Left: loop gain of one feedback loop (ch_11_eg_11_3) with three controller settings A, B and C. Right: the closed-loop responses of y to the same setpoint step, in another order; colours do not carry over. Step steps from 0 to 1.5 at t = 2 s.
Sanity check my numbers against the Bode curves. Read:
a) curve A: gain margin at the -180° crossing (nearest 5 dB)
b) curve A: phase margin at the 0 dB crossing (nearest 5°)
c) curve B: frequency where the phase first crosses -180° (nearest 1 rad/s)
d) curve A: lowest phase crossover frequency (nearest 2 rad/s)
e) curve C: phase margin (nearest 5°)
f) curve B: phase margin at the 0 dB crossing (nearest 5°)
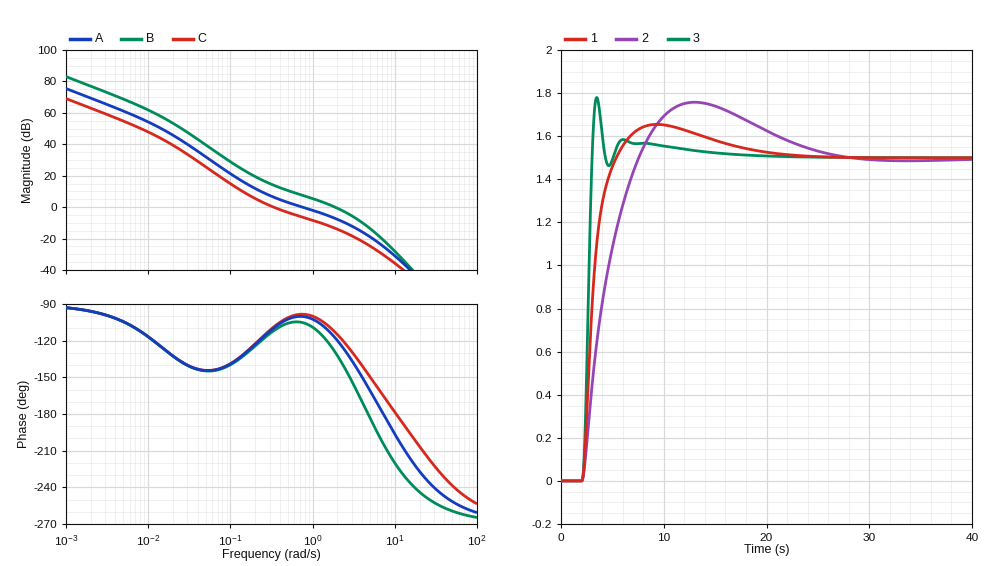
25 dB
80°
5 rad/s
8 rad/s
70°
50°
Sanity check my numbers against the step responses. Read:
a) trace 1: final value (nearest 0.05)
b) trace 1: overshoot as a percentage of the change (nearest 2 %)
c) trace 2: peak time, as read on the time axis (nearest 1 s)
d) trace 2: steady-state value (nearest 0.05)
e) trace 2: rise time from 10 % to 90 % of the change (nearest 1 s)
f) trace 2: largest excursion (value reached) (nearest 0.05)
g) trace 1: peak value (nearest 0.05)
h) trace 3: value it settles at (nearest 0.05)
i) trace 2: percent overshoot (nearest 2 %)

1.50
10 %
13 s
1.50
4 s
1.75
1.65
1.50
18 %
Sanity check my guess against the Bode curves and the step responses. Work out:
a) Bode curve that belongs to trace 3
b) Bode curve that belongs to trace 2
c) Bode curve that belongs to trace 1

B
C
A
